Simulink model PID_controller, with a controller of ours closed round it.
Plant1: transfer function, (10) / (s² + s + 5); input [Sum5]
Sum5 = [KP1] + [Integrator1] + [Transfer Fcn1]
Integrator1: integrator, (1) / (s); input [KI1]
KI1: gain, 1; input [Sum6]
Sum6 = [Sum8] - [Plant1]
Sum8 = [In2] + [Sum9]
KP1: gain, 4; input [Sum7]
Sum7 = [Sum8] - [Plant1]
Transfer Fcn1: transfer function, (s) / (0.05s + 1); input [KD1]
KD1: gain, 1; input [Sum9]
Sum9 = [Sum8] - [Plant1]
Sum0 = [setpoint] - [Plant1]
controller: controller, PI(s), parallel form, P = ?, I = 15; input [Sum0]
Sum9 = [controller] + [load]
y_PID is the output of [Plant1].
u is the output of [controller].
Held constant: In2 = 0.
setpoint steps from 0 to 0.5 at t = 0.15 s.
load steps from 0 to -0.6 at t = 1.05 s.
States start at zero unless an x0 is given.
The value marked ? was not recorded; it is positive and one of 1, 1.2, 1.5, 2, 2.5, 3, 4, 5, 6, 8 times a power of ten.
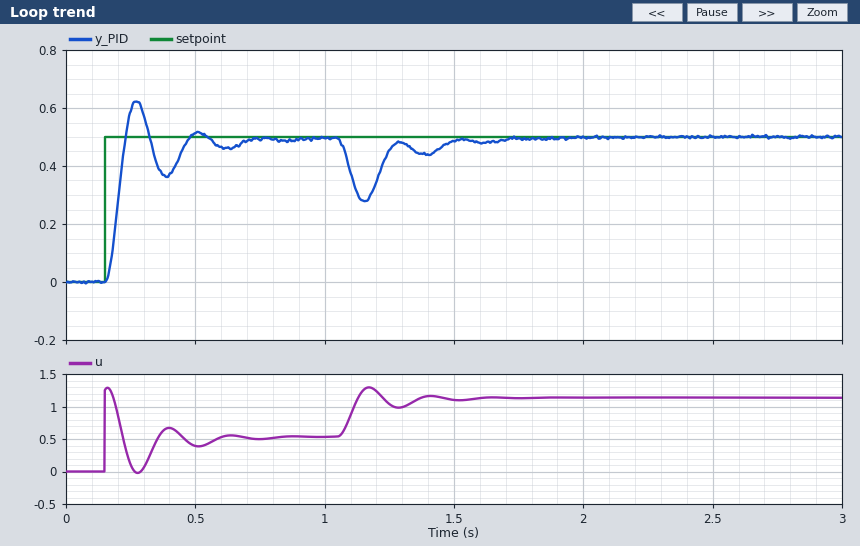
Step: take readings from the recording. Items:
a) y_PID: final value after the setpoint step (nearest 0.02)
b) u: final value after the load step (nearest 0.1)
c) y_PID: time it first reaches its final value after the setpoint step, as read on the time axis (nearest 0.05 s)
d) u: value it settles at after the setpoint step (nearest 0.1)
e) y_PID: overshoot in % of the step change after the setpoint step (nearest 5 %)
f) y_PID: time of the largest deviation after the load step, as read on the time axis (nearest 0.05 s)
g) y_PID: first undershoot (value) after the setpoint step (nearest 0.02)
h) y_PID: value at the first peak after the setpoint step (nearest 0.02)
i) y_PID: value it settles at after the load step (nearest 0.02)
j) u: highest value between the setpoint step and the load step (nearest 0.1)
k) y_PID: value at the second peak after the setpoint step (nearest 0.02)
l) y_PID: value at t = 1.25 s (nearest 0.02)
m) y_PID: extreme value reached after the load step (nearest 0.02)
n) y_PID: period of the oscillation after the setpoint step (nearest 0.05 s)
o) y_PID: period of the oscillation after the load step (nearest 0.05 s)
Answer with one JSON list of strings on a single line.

["0.50", "1.1", "0.25 s", "0.5", "25 %", "1.15 s", "0.36", "0.62", "0.50", "1.3", "0.52", "0.46", "0.28", "0.25 s", "0.25 s"]
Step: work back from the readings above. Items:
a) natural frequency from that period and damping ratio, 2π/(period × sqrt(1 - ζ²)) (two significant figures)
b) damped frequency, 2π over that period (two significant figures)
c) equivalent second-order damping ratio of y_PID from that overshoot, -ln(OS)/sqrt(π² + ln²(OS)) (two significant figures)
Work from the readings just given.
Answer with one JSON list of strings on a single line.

["27 rad/s", "25 rad/s", "0.40"]
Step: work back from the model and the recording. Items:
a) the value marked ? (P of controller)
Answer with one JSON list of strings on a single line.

["2.5"]
